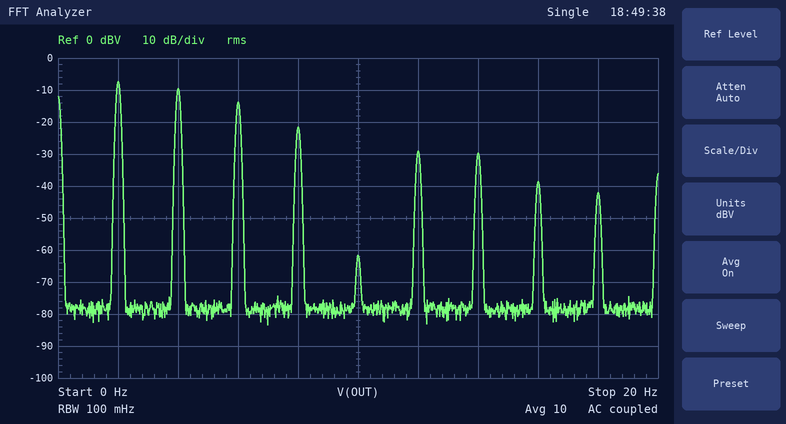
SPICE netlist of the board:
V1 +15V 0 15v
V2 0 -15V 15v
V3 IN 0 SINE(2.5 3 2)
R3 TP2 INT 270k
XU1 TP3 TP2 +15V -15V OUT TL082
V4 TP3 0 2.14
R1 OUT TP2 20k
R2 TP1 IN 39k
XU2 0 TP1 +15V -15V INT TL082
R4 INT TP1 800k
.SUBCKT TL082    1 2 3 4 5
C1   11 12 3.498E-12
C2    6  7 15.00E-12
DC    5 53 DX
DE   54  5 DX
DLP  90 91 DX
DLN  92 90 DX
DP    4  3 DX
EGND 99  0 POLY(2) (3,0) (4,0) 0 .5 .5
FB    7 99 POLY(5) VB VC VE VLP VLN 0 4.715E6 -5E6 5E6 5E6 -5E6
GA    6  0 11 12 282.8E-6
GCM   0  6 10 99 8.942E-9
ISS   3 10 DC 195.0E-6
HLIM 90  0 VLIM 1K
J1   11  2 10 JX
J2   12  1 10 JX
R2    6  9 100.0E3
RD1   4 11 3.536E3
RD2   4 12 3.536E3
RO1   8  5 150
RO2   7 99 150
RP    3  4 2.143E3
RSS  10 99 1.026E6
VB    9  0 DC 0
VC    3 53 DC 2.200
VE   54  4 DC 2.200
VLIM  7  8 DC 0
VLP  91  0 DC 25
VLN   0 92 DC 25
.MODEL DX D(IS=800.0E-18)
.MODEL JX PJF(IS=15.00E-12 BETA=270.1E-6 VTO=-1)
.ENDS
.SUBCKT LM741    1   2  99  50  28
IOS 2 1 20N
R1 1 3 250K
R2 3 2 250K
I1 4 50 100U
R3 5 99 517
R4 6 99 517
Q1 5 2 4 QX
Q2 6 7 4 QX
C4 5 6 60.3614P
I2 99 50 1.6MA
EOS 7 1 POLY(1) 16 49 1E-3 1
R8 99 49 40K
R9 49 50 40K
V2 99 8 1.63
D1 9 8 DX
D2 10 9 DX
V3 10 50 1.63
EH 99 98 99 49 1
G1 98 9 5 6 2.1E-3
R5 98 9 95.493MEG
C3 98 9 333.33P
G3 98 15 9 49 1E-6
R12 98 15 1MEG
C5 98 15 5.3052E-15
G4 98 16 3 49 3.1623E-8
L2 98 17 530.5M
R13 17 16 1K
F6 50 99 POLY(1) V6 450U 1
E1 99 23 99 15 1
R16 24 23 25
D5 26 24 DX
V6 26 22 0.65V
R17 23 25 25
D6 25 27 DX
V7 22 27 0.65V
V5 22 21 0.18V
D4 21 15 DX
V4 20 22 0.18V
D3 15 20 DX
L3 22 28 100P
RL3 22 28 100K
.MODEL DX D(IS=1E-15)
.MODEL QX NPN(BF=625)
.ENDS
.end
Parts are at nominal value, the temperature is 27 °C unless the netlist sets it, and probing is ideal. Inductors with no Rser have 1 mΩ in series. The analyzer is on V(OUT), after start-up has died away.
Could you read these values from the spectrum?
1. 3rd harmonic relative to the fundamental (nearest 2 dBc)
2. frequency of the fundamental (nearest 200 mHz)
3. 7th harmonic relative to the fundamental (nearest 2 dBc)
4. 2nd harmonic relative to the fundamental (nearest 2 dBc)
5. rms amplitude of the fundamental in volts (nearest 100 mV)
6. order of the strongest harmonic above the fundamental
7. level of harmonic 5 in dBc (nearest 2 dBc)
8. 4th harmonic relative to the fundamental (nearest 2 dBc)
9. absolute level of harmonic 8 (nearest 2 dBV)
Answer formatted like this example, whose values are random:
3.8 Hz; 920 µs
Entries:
-6 dBc; 2.0 Hz; -22 dBc; -2 dBc; 400 mV; 2; -54 dBc; -14 dBc; -38 dBV
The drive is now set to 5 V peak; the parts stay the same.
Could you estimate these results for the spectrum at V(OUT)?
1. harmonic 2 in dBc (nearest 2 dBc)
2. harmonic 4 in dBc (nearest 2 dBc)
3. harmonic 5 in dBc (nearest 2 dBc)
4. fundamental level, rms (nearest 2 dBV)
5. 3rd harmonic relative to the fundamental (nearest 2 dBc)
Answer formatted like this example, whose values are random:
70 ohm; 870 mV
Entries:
-6 dBc; -12 dBc; -14 dBc; -2 dBV; -52 dBc
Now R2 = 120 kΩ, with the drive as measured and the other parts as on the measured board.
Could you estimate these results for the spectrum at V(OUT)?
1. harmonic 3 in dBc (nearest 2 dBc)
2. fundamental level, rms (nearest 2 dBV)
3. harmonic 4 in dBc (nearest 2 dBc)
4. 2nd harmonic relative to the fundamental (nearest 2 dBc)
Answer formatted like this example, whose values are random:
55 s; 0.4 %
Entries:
-22 dBc; -8 dBV; -22 dBc; -6 dBc
